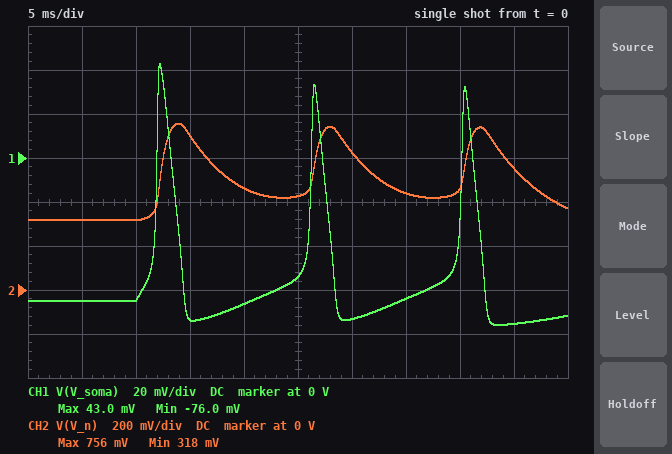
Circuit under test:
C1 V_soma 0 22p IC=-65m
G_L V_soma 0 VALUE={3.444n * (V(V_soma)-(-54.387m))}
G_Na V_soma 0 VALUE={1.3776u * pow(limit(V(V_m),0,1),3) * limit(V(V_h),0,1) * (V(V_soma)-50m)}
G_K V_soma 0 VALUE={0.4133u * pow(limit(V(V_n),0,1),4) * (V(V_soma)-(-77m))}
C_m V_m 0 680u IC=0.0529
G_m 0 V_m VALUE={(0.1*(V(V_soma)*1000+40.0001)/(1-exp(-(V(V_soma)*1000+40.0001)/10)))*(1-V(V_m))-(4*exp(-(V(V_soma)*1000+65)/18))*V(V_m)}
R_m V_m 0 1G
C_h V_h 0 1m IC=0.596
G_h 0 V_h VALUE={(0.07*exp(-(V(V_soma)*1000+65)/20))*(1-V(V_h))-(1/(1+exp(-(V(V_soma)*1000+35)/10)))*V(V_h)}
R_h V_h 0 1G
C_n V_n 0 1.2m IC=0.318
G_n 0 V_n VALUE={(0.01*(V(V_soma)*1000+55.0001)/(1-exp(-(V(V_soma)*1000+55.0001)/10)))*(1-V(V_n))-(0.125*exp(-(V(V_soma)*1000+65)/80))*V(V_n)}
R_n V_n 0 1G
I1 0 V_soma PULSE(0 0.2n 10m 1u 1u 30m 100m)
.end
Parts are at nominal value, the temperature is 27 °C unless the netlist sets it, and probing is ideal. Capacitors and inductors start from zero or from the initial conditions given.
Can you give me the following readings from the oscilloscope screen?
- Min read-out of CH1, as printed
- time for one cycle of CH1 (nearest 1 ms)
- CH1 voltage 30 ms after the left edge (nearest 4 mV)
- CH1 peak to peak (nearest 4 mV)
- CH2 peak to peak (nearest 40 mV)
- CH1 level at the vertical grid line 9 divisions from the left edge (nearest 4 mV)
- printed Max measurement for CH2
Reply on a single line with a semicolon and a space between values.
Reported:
-76.0 mV; 14 ms; -72 mV; 120 mV; 440 mV; -76 mV; 756 mV
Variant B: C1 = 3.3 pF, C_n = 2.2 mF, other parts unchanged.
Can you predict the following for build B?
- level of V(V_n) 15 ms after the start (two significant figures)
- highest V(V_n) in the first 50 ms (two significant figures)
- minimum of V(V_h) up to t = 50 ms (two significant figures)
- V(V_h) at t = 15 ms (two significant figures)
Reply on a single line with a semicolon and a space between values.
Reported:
620 mV; 690 mV; 52 mV; 200 mV
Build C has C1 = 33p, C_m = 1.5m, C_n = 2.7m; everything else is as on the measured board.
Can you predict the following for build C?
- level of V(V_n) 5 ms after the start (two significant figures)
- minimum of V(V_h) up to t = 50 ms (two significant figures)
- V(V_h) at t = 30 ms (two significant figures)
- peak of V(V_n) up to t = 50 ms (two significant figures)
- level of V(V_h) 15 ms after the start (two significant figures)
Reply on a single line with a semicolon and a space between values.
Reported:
320 mV; 31 mV; 530 mV; 660 mV; 61 mV
